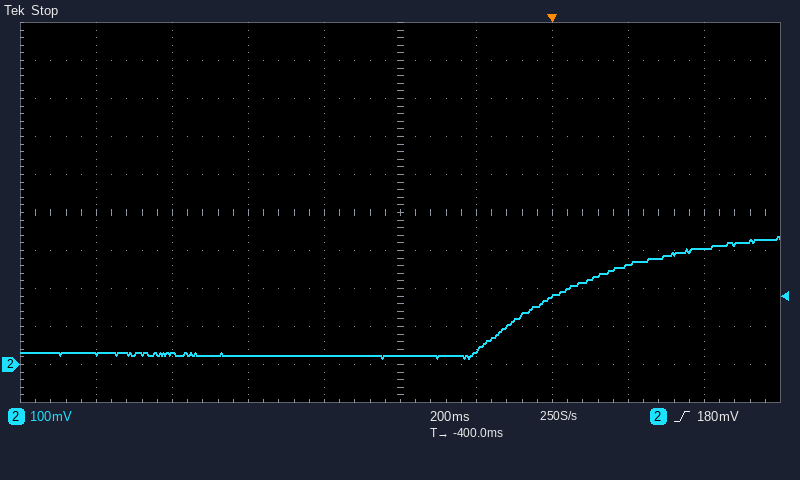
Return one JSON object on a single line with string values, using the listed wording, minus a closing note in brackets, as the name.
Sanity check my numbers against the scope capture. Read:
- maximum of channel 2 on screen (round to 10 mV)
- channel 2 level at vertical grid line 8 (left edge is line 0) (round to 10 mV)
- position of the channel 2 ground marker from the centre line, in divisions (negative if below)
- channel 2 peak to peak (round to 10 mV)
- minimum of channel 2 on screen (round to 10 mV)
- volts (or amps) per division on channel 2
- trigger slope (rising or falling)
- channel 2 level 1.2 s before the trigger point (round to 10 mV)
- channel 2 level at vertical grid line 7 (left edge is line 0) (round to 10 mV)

{"maximum of channel 2 on screen": "340 mV", "channel 2 level at vertical grid line 8 (left edge is line 0)": "260 mV", "position of the channel 2 ground marker from the centre line, in divisions": "-4.0 div", "channel 2 peak to peak": "320 mV", "minimum of channel 2 on screen": "20 mV", "volts (or amps) per division on channel 2": "100 mV", "trigger slope": "rising", "channel 2 level 1.2 s before the trigger point": "30 mV", "channel 2 level at vertical grid line 7 (left edge is line 0)": "180 mV"}
